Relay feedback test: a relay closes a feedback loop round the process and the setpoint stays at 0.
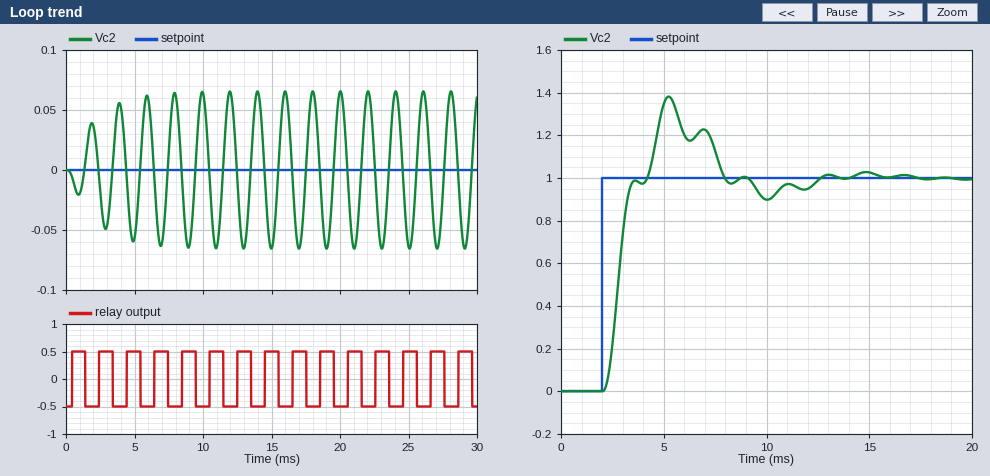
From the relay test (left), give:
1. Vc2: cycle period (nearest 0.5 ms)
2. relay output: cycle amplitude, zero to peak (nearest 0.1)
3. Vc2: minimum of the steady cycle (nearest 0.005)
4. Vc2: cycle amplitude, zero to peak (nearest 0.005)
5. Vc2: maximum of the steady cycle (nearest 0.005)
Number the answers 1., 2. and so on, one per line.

1. 2.0 ms
2. 0.5
3. -0.065
4. 0.065
5. 0.065
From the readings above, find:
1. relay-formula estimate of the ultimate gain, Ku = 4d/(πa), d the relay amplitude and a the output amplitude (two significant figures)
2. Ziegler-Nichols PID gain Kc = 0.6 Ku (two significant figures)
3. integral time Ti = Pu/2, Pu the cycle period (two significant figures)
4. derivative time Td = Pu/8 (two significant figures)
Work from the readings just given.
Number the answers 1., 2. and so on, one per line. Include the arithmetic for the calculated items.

1. 4 × 0.5 / (π × 0.065) = 9.8
2. 0.6 × 9.8 = 5.9
3. 2 / 2 = 1.0 ms
4. 2 / 8 = 0.25 ms
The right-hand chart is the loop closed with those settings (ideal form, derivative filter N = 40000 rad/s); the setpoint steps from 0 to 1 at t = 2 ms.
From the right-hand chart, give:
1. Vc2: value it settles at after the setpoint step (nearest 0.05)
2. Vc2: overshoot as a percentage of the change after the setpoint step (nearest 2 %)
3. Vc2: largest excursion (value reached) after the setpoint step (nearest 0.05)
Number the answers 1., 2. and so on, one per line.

1. 1.00
2. 38 %
3. 1.40
